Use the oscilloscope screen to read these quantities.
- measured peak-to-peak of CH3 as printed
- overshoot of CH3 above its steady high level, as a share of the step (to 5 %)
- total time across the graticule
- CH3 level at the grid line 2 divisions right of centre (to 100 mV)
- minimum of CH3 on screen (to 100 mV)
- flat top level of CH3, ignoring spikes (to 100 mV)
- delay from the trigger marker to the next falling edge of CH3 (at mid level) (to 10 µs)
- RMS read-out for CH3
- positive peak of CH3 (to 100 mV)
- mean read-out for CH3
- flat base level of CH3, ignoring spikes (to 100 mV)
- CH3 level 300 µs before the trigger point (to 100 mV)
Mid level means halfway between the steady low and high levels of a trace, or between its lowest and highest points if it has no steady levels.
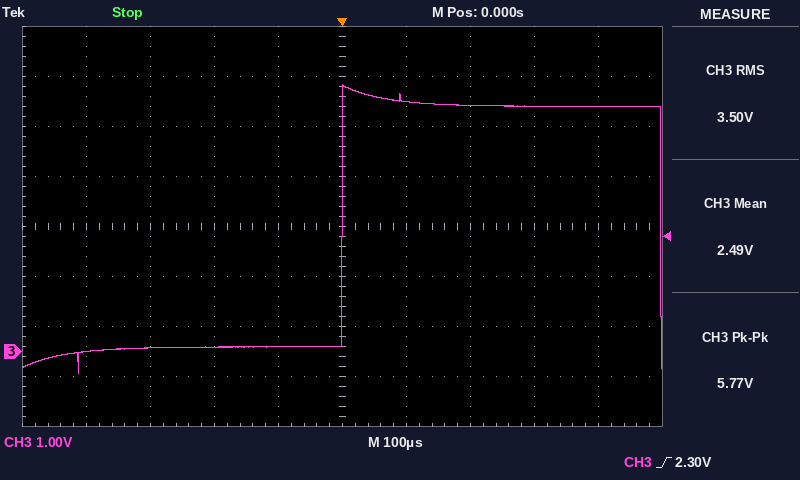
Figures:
5.77 V
10 %
1 ms
4.9 V
-400 mV
4.9 V
500 µs
3.50 V
5.3 V
2.49 V
100 mV
100 mV
